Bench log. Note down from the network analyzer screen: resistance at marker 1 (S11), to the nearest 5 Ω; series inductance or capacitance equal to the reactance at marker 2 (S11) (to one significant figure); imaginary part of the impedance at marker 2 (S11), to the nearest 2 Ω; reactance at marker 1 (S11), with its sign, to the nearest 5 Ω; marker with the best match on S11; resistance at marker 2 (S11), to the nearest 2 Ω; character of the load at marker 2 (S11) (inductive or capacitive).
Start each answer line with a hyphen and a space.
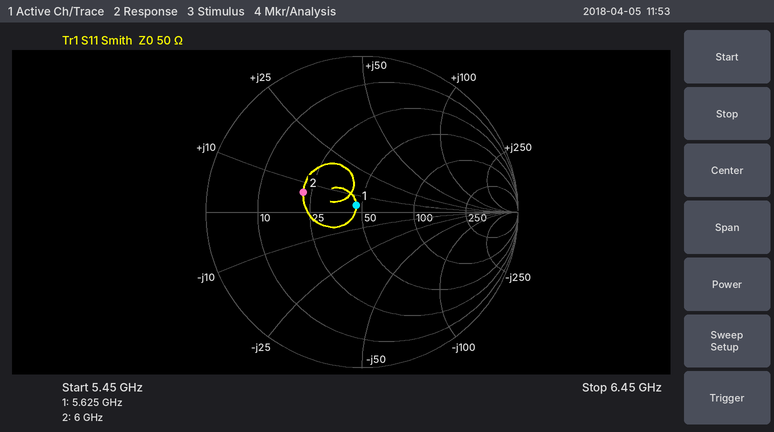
- 45 Ω
- 200 pH
- +6 Ω
- +5 Ω
- marker 1
- 22 Ω
- inductive
